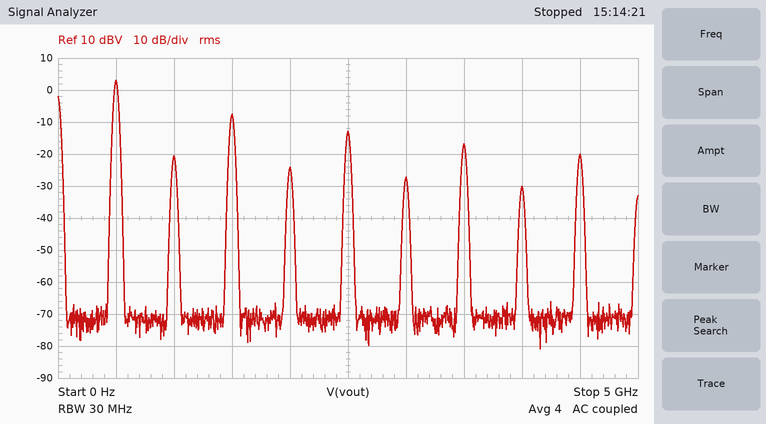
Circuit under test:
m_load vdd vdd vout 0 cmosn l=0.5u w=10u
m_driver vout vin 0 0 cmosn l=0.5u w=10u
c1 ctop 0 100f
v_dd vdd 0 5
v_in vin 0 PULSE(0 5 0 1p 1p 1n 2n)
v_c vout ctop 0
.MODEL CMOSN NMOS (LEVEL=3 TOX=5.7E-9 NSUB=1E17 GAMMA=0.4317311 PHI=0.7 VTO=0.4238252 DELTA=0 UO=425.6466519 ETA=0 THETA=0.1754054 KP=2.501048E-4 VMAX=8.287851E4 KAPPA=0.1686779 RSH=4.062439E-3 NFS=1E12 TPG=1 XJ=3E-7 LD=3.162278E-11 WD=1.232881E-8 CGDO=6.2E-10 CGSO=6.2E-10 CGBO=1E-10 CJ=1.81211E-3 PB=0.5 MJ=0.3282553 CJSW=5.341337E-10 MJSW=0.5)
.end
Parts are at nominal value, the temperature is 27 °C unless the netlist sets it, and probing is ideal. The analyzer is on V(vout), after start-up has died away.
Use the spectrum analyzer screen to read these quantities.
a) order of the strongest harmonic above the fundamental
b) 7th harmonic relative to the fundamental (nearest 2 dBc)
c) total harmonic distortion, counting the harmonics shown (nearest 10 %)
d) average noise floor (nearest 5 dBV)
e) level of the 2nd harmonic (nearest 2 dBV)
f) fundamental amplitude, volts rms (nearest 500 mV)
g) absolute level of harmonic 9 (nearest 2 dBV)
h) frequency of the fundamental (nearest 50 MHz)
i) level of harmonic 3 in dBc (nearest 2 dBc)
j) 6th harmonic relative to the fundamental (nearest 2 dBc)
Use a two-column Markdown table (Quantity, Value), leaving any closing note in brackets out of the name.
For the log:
| Quantity | Value |
|---|---|
| order of the strongest harmonic above the fundamental | 3 |
| 7th harmonic relative to the fundamental | -20 dBc |
| total harmonic distortion, counting the harmonics shown | 40 % |
| average noise floor | -70 dBV |
| level of the 2nd harmonic | -20 dBV |
| fundamental amplitude, volts rms | 1.5 V |
| absolute level of harmonic 9 | -20 dBV |
| frequency of the fundamental | 500 MHz |
| level of harmonic 3 in dBc | -10 dBc |
| 6th harmonic relative to the fundamental | -30 dBc |
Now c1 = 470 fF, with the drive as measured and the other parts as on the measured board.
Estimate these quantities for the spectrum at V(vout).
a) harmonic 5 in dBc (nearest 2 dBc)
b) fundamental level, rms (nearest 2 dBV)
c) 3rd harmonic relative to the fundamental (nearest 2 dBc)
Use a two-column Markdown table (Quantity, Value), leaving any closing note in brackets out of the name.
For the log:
| Quantity | Value |
|---|---|
| harmonic 5 in dBc | -22 dBc |
| fundamental level, rms | 2 dBV |
| 3rd harmonic relative to the fundamental | -14 dBc |
